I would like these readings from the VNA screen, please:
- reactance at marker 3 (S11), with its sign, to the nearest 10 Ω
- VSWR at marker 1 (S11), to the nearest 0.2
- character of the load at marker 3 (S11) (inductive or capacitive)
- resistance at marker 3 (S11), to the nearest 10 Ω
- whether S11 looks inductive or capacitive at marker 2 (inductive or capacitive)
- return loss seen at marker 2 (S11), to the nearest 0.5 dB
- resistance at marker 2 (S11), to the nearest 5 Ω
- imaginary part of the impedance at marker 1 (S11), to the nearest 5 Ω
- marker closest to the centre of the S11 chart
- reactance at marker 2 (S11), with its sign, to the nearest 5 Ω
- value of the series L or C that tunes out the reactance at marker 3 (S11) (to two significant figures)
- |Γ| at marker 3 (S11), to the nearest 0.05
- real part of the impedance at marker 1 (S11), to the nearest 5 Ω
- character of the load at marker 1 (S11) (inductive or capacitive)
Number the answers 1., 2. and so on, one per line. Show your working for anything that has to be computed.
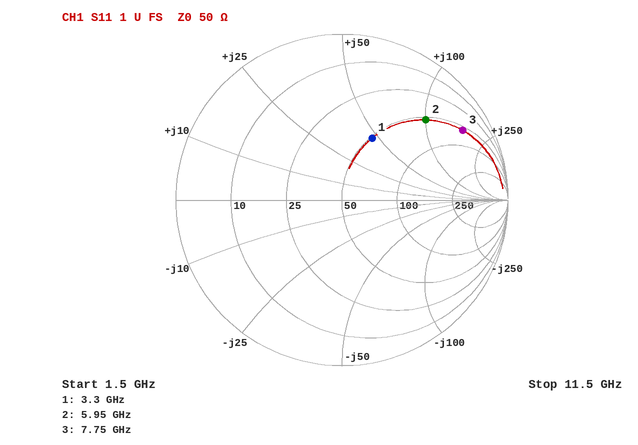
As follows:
1. +170 Ω
2. 2.4
3. inductive
4. 60 Ω
5. inductive
6. 3.0 dB
7. 55 Ω
8. +45 Ω
9. marker 1
10. +100 Ω
11. C = 1/(2π × 7.75 GHz × 170 Ω) ≈ 121 fF, so 120 fF to two significant figures
12. 0.85
13. 50 Ω
14. inductive
